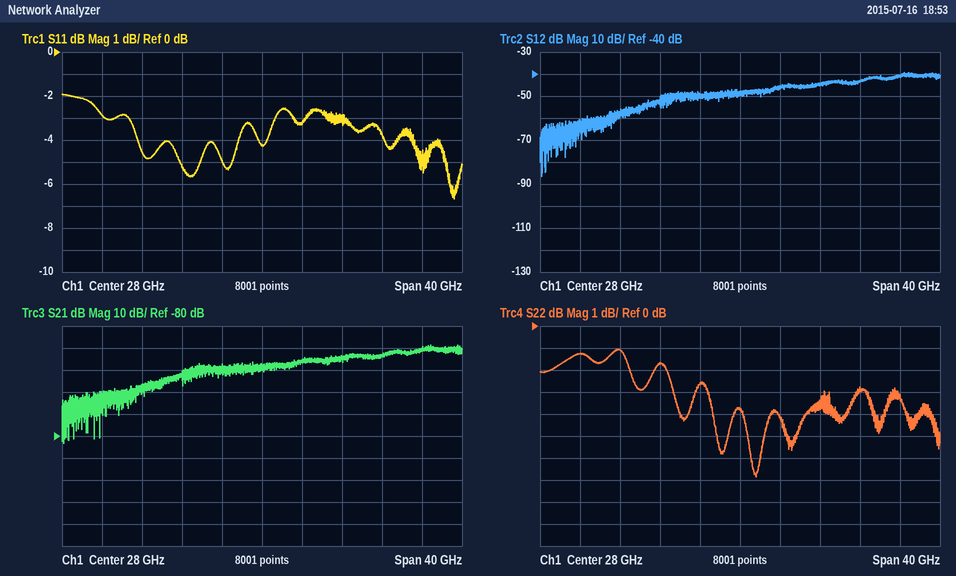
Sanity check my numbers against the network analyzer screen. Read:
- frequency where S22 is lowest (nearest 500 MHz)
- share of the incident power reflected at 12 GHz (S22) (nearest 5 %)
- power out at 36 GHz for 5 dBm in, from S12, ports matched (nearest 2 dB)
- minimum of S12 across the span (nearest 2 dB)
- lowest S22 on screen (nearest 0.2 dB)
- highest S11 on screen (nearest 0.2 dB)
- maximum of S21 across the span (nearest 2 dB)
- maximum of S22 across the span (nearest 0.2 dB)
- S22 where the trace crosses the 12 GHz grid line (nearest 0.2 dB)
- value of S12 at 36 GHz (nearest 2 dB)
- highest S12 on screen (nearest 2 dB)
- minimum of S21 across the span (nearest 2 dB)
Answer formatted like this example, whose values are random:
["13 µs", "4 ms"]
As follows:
["29.5 GHz", "75 %", "-40 dBm", "-86 dB", "-6.8 dB", "-2.0 dB", "-38 dB", "-1.0 dB", "-1.2 dB", "-44 dB", "-40 dB", "-84 dB"]
